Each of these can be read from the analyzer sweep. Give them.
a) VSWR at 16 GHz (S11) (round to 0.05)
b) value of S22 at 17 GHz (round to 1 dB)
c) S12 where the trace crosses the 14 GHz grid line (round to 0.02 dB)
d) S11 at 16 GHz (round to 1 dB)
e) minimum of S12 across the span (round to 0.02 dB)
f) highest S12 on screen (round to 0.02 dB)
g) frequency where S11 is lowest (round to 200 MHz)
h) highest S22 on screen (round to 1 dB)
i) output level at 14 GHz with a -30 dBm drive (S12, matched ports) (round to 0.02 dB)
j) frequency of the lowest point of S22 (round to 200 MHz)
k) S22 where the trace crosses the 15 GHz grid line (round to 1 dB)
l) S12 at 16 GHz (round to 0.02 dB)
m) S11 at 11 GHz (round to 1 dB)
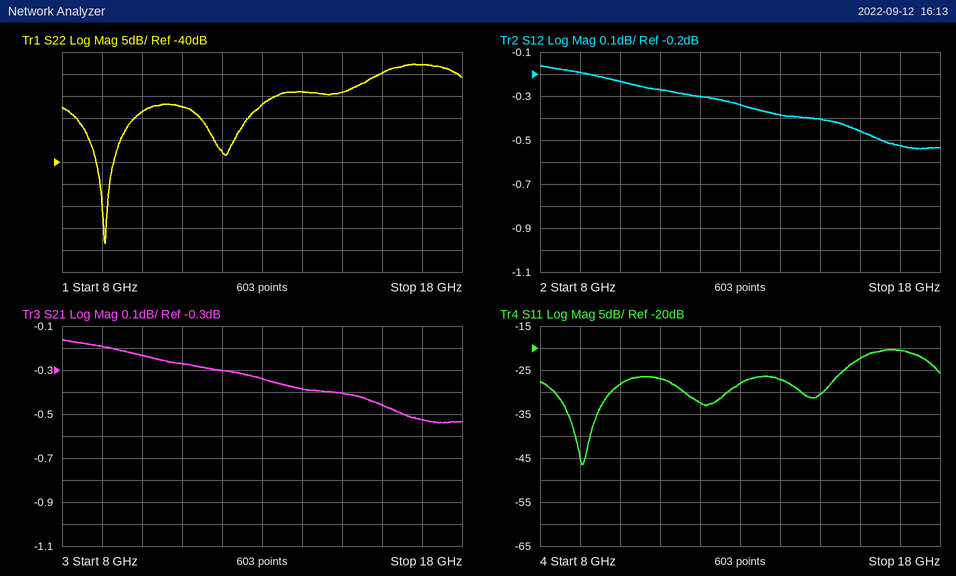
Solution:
1.15
-18 dB
-0.38 dB
-22 dB
-0.54 dB
-0.16 dB
9.0 GHz
-18 dB
-30.38 dBm
9.0 GHz
-24 dB
-0.46 dB
-27 dB
